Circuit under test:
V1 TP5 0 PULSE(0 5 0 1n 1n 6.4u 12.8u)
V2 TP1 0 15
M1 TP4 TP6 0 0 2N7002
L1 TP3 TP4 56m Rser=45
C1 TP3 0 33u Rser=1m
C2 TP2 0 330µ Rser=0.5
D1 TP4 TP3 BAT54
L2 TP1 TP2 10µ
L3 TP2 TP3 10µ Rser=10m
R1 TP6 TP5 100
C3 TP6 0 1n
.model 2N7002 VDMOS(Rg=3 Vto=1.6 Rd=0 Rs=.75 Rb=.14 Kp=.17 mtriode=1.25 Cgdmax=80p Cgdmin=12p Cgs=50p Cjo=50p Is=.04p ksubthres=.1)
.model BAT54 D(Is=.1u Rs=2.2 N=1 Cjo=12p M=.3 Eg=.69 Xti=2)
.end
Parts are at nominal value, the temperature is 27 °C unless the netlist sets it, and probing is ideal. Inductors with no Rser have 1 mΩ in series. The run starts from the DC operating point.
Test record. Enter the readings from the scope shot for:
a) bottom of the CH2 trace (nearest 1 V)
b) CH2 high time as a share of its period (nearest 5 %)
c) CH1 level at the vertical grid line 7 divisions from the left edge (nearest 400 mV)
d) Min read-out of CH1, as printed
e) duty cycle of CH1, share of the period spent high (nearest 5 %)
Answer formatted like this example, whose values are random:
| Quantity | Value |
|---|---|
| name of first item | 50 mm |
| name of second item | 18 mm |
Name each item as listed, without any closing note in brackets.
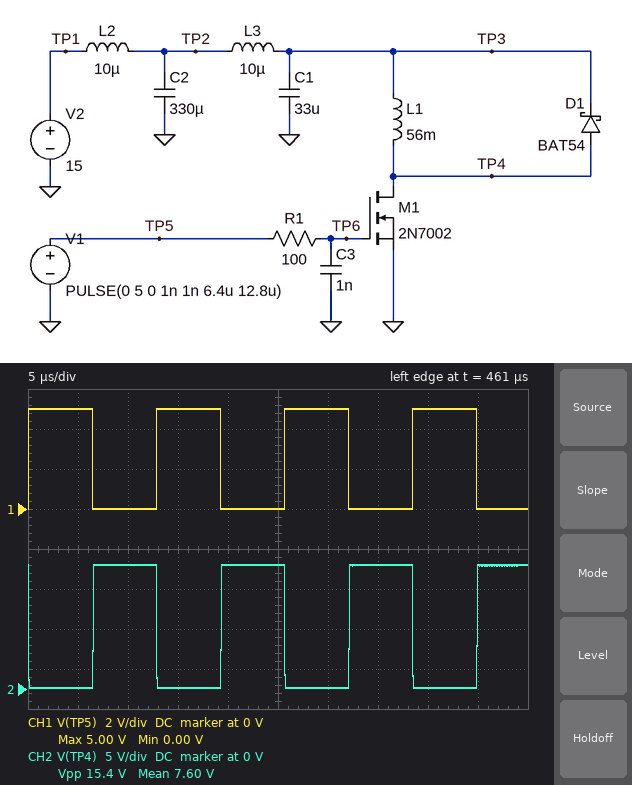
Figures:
| Quantity | Value |
|---|---|
| bottom of the CH2 trace | 0 V |
| CH2 high time as a share of its period | 50 % |
| CH1 level at the vertical grid line 7 divisions from the left edge | 0 V |
| Min read-out of CH1, as printed | 0.00 V |
| duty cycle of CH1, share of the period spent high | 50 % |
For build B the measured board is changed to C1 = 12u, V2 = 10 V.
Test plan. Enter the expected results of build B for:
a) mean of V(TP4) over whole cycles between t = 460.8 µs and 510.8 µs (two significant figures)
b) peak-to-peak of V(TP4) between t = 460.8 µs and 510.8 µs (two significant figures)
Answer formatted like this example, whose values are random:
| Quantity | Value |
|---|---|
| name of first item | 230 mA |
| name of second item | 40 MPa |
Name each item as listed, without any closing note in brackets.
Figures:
| Quantity | Value |
|---|---|
| mean of V(TP4) over whole cycles between t = 460.8 µs and 510.8 µs | 5.2 V |
| peak-to-peak of V(TP4) between t = 460.8 µs and 510.8 µs | 10 V |
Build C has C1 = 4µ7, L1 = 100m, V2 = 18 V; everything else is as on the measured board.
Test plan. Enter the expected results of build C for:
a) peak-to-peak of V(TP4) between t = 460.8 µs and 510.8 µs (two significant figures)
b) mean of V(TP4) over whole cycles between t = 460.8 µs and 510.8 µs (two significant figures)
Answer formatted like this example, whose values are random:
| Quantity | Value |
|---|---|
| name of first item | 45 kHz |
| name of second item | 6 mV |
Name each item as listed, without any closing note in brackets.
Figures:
| Quantity | Value |
|---|---|
| peak-to-peak of V(TP4) between t = 460.8 µs and 510.8 µs | 18 V |
| mean of V(TP4) over whole cycles between t = 460.8 µs and 510.8 µs | 9.2 V |
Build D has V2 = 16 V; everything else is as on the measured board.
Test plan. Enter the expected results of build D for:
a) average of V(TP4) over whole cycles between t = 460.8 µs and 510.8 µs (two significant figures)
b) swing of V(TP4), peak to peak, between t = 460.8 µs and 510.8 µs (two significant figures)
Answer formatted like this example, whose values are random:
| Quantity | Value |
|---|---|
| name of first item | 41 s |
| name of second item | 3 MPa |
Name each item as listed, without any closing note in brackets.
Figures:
| Quantity | Value |
|---|---|
| average of V(TP4) over whole cycles between t = 460.8 µs and 510.8 µs | 8.3 V |
| swing of V(TP4), peak to peak, between t = 460.8 µs and 510.8 µs | 16 V |
